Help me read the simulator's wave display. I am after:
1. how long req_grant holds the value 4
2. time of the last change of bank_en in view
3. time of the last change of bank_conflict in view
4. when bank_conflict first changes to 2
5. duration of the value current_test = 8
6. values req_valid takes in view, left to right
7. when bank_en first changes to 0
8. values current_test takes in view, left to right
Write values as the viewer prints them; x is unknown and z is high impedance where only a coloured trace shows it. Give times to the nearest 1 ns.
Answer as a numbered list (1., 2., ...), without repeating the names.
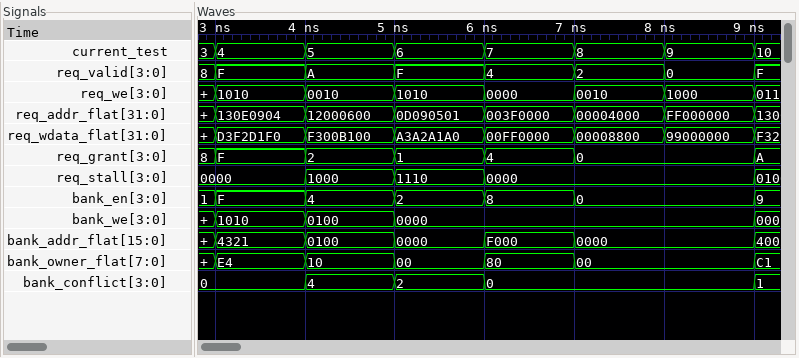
1. 1 ns
2. 9 ns
3. 9 ns
4. 5 ns
5. 1 ns
6. 8, F, A, F, 4, 2, 0, F
7. 7 ns
8. 3, 4, 5, 6, 7, 8, 9, 10
